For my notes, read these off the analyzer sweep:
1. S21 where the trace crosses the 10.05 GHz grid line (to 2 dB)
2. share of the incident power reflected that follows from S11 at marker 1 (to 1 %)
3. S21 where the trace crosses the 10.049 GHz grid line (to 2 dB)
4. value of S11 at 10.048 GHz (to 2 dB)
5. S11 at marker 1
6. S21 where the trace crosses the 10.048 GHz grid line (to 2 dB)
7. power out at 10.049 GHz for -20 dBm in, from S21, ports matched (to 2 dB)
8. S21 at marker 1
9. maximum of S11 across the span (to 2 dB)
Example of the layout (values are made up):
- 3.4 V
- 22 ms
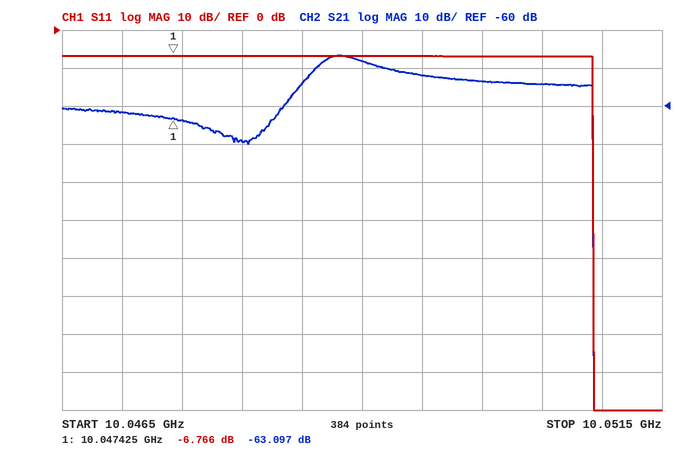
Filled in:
- -54 dB
- 21 %
- -48 dB
- -6 dB
- -6.766 dB
- -70 dB
- -68 dBm
- -63.097 dB
- -6 dB
